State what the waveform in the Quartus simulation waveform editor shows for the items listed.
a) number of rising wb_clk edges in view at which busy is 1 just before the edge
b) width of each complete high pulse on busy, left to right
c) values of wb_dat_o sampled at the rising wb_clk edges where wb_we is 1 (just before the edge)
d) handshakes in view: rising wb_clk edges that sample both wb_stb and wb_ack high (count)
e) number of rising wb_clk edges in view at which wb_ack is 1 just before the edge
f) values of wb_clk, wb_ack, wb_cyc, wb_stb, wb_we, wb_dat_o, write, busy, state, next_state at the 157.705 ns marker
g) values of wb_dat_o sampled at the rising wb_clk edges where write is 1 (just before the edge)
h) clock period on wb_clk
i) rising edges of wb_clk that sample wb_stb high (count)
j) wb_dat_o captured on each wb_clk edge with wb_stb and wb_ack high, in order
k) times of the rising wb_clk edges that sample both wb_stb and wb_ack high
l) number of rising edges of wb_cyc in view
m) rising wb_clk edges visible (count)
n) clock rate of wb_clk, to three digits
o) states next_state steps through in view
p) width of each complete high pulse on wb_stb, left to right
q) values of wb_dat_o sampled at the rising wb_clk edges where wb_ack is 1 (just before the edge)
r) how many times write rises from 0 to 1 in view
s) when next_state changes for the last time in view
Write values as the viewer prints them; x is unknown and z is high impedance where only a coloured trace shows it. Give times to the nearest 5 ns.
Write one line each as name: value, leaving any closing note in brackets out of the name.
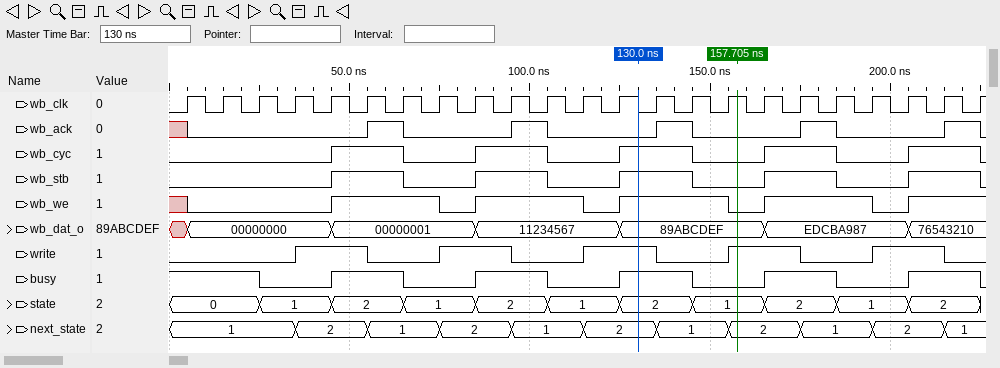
number of rising wb_clk edges in view at which busy is 1 just before the edge: 13
width of each complete high pulse on busy, left to right: 20 ns, 20 ns, 20 ns, 20 ns, 20 ns
values of wb_dat_o sampled at the rising wb_clk edges where wb_we is 1: 00000001, 00000001, 00000001, 11234567, 11234567, 11234567, 89ABCDEF, 89ABCDEF, 89ABCDEF, EDCBA987, EDCBA987, EDCBA987, 76543210, 76543210
handshakes in view: rising wb_clk edges that sample both wb_stb and wb_ack high: 5
number of rising wb_clk edges in view at which wb_ack is 1 just before the edge: 5
values of wb_clk, wb_ack, wb_cyc, wb_stb, wb_we, wb_dat_o, write, busy, state, next_state at the 157.705 ns marker: wb_clk=1, wb_ack=0, wb_cyc=0, wb_stb=0, wb_we=0, wb_dat_o=89ABCDEF, write=1, busy=0, state=1, next_state=2
values of wb_dat_o sampled at the rising wb_clk edges where write is 1: 00000000, 00000001, 00000001, 11234567, 11234567, 89ABCDEF, 89ABCDEF, EDCBA987, EDCBA987, 76543210
clock period on wb_clk: 10 ns
rising edges of wb_clk that sample wb_stb high: 10
wb_dat_o captured on each wb_clk edge with wb_stb and wb_ack high, in order: 00000001, 11234567, 89ABCDEF, EDCBA987, 76543210
times of the rising wb_clk edges that sample both wb_stb and wb_ack high: 65 ns, 105 ns, 145 ns, 185 ns, 225 ns
number of rising edges of wb_cyc in view: 5
rising wb_clk edges visible: 23
clock rate of wb_clk, to three digits: 100 MHz
states next_state steps through in view: 1, 2, 1, 2, 1, 2, 1, 2, 1, 2, 1
width of each complete high pulse on wb_stb, left to right: 20 ns, 20 ns, 20 ns, 20 ns, 20 ns
values of wb_dat_o sampled at the rising wb_clk edges where wb_ack is 1: 00000001, 11234567, 89ABCDEF, EDCBA987, 76543210
how many times write rises from 0 to 1 in view: 5
when next_state changes for the last time in view: 215 ns
